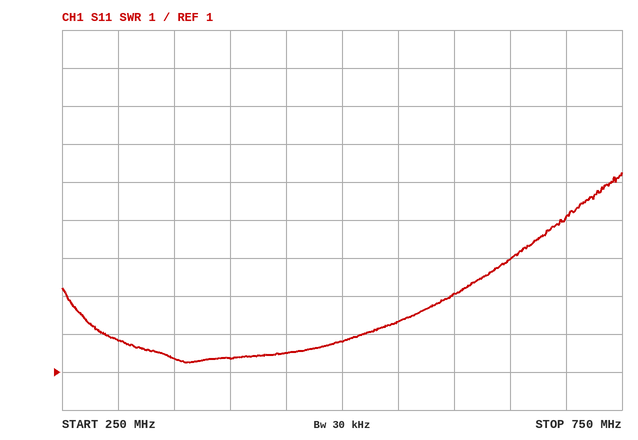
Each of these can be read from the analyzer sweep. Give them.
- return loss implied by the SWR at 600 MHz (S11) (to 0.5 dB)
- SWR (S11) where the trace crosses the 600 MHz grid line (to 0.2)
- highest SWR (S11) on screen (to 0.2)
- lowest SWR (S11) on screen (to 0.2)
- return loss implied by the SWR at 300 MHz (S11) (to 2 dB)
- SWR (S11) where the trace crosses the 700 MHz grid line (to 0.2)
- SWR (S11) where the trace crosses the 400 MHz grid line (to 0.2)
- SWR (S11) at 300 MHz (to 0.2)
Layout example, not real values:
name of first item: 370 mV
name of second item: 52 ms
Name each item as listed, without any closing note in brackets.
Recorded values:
return loss implied by the SWR at 600 MHz (S11): 6.0 dB
SWR (S11) where the trace crosses the 600 MHz grid line: 3.0
highest SWR (S11) on screen: 6.2
lowest SWR (S11) on screen: 1.2
return loss implied by the SWR at 300 MHz (S11): 10 dB
SWR (S11) where the trace crosses the 700 MHz grid line: 5.0
SWR (S11) where the trace crosses the 400 MHz grid line: 1.4
SWR (S11) at 300 MHz: 1.8
